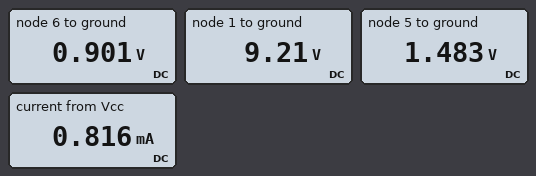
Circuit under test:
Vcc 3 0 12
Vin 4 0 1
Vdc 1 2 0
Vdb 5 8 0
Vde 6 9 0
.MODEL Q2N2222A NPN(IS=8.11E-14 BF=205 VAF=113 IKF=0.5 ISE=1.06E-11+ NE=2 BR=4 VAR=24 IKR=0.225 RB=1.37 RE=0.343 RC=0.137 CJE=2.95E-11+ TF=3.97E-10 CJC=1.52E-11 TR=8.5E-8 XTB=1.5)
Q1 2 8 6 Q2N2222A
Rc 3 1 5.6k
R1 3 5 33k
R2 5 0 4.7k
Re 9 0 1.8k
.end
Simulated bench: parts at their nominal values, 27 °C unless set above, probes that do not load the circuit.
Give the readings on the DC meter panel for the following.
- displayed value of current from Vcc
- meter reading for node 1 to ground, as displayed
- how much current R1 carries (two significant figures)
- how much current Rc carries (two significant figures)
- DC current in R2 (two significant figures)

0.816 mA
9.21 V
320 µA
500 µA
320 µA
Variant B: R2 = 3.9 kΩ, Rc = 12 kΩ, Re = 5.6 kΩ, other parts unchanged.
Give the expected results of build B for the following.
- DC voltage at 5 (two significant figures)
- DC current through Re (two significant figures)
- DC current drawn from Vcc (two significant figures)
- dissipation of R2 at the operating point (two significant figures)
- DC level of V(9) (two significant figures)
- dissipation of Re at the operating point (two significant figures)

1.3 V
130 µA
450 µA
410 µW
720 mV
92 µW
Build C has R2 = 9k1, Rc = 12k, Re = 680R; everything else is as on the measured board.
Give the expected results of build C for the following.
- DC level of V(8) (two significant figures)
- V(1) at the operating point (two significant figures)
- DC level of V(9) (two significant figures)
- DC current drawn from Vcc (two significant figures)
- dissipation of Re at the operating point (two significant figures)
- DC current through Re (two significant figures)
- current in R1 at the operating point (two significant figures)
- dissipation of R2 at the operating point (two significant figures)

1.4 V
780 mV
750 mV
1.3 mA
830 µW
1.1 mA
320 µA
210 µW
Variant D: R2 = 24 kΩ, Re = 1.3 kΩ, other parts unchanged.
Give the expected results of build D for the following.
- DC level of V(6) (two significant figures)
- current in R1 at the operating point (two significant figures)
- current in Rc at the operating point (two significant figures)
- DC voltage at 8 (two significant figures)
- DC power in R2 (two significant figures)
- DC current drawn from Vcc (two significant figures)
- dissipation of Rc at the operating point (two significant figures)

2.4 V
270 µA
1.7 mA
3.0 V
380 µW
2.0 mA
16 mW
